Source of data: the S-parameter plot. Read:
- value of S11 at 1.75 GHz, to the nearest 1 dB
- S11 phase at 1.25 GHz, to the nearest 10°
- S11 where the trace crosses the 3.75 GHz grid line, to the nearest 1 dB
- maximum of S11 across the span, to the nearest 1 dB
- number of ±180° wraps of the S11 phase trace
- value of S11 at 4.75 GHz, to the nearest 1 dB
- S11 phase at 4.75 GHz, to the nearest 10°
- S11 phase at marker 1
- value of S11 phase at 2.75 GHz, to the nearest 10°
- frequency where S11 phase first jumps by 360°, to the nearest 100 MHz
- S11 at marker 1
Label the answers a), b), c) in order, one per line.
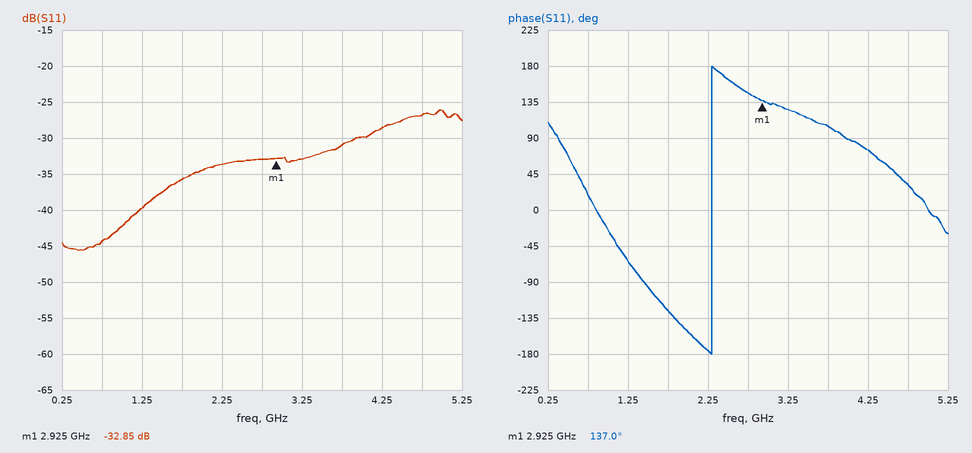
a) -36 dB
b) -60°
c) -31 dB
d) -26 dB
e) 1
f) -27 dB
g) 30°
h) 137.0°
i) 150°
j) 2.3 GHz
k) -32.85 dB
